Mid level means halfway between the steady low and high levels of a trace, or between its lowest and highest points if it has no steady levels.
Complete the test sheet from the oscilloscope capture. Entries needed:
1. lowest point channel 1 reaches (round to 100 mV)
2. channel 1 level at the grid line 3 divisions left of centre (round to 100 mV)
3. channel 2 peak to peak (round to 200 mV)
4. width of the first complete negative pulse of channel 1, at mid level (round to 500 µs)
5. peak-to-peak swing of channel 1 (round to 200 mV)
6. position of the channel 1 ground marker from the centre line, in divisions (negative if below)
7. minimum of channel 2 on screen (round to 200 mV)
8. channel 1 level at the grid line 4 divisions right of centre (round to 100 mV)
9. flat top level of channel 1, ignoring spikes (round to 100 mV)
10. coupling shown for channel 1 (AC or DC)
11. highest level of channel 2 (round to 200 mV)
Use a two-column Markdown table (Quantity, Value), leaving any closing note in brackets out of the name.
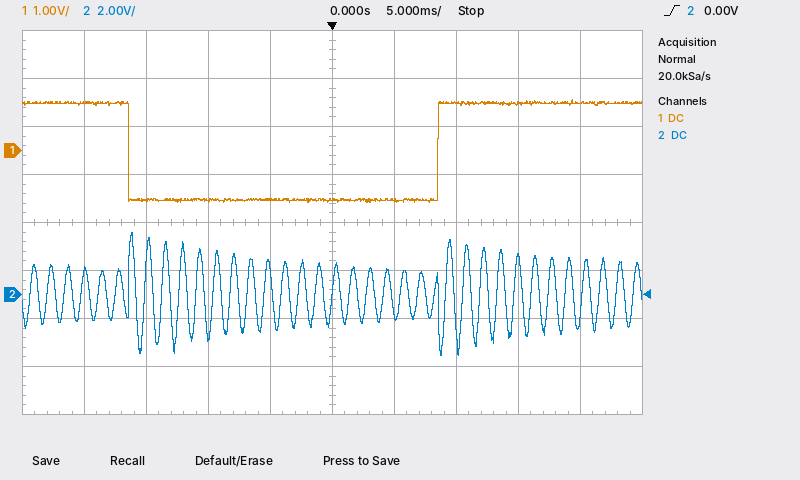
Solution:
| Quantity | Value |
|---|---|
| lowest point channel 1 reaches | -1.1 V |
| channel 1 level at the grid line 3 divisions left of centre | -1.0 V |
| channel 2 peak to peak | 5.2 V |
| width of the first complete negative pulse of channel 1, at mid level | 25.0 ms |
| peak-to-peak swing of channel 1 | 2.2 V |
| position of the channel 1 ground marker from the centre line, in divisions | +1.5 div |
| minimum of channel 2 on screen | -2.6 V |
| channel 1 level at the grid line 4 divisions right of centre | 1.0 V |
| flat top level of channel 1, ignoring spikes | 1.0 V |
| coupling shown for channel 1 | DC |
| highest level of channel 2 | 2.6 V |
